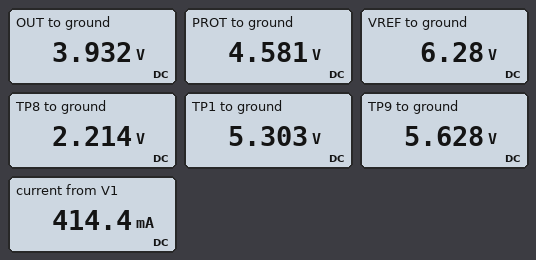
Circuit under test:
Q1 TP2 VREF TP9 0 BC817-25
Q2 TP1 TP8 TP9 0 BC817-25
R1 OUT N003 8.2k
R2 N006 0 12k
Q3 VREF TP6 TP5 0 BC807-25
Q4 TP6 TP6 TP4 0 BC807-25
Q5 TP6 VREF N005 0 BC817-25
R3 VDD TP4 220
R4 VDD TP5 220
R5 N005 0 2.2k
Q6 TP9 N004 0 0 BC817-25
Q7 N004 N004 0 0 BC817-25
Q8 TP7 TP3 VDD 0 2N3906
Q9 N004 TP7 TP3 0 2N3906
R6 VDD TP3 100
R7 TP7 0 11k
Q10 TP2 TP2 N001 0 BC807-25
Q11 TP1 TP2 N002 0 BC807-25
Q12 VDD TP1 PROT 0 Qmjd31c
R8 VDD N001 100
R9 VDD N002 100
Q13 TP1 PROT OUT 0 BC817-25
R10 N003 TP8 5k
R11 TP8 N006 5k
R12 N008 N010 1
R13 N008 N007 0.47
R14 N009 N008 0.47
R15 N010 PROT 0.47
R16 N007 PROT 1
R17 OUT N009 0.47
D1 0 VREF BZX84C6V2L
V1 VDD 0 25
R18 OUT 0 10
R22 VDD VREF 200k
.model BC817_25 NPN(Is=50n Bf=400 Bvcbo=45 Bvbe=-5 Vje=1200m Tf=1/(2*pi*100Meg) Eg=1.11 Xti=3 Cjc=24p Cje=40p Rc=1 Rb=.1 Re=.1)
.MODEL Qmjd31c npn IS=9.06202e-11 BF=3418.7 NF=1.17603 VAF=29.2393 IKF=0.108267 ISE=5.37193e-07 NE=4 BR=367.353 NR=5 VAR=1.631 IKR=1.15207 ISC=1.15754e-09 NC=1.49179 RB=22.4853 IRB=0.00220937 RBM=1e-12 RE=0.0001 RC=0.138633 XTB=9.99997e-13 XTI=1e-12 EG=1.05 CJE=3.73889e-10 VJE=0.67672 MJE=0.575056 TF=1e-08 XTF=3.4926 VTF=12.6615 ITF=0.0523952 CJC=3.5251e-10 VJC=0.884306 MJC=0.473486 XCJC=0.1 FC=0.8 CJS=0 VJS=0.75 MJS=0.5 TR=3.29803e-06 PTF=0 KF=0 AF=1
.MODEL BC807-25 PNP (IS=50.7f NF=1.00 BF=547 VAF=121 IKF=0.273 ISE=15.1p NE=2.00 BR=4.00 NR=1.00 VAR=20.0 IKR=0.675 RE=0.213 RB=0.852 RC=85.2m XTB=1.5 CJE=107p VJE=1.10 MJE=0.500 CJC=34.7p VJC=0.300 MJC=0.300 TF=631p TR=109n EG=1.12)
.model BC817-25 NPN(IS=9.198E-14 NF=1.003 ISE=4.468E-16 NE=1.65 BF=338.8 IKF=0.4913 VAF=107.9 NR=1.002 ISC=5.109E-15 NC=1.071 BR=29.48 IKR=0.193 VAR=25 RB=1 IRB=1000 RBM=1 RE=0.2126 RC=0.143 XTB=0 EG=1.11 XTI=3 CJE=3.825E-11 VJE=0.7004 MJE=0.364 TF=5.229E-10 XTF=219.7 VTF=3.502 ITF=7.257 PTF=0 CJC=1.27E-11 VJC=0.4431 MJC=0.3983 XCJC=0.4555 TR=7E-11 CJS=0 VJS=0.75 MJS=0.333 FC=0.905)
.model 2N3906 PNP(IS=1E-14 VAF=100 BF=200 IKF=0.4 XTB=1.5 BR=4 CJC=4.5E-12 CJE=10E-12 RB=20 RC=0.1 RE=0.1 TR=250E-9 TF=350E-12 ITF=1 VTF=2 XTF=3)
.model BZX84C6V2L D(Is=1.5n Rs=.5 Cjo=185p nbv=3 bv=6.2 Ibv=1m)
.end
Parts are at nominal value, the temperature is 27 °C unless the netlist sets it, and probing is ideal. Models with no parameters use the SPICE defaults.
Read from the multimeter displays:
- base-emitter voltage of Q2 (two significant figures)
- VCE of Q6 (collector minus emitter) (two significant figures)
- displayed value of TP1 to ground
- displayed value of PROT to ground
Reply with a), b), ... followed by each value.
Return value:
a) -3.4 V
b) 5.6 V
c) 5.303 V
d) 4.581 V
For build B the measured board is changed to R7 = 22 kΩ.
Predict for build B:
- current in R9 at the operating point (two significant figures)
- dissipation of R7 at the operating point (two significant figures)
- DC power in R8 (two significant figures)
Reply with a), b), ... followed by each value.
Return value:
a) 6.8 mA
b) 25 mW
c) 4.6 mW
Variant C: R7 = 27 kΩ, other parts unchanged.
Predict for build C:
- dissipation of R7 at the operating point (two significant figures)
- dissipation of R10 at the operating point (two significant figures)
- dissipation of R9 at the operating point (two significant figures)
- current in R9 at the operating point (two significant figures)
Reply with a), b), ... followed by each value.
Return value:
a) 21 mW
b) 84 µW
c) 4.5 mW
d) 6.7 mA
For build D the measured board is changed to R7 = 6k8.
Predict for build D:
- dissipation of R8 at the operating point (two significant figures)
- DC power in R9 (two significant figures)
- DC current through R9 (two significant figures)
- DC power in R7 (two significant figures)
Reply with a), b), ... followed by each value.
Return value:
a) 5.0 mW
b) 5.1 mW
c) 7.1 mA
d) 82 mW
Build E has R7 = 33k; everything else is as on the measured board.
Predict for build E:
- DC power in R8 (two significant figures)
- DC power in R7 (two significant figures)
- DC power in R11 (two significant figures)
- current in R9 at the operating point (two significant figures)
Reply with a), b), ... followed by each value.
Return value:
a) 4.4 mW
b) 17 mW
c) 84 µW
d) 6.7 mA
